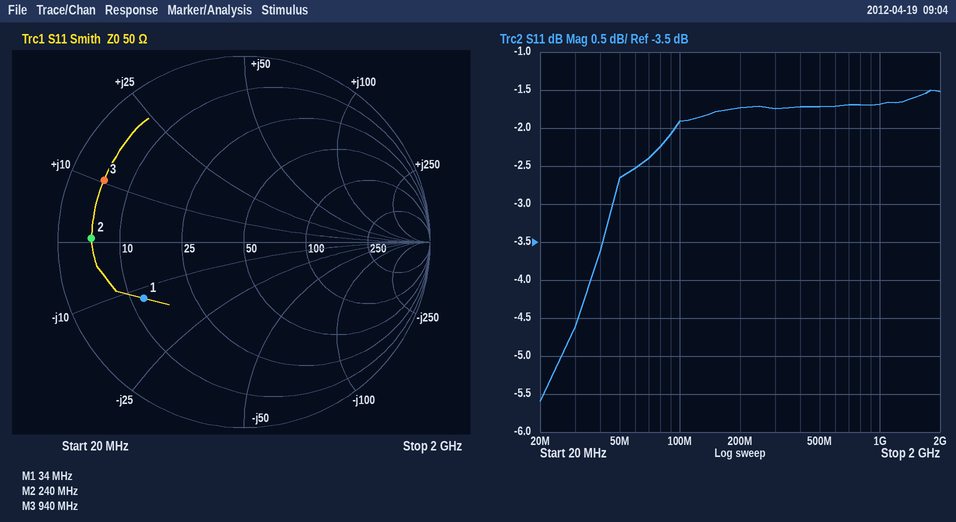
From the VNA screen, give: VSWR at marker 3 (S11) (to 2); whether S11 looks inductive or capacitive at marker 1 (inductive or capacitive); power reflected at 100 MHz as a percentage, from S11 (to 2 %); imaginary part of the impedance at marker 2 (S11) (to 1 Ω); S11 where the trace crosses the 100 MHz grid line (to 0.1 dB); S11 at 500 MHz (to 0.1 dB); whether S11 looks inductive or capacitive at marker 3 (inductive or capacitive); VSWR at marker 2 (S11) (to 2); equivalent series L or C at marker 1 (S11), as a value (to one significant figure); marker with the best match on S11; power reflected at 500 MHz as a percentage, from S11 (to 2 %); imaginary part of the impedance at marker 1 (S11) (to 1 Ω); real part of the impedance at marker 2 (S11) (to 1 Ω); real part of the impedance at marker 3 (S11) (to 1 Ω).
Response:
10
capacitive
64 %
+1 Ω
-1.9 dB
-1.7 dB
inductive
10
400 pF
marker 1
68 %
-12 Ω
5 Ω
5 Ω
